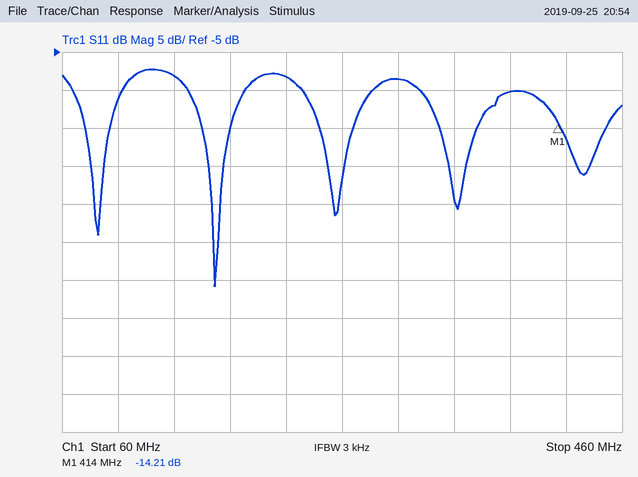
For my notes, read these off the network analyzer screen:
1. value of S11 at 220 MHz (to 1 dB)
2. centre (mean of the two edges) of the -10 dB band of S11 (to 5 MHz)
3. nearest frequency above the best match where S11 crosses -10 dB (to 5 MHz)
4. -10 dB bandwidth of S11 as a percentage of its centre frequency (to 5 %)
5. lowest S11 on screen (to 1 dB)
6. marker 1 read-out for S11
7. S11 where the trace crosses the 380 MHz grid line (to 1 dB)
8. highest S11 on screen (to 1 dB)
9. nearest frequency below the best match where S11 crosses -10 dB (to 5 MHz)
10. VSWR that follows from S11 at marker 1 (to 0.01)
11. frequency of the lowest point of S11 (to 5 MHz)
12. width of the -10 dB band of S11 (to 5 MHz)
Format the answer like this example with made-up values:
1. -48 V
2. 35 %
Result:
1. -8 dB
2. 170 MHz
3. 190 MHz
4. 25 %
5. -36 dB
6. -14.21 dB
7. -10 dB
8. -7 dB
9. 150 MHz
10. 1.48
11. 170 MHz
12. 40 MHz
